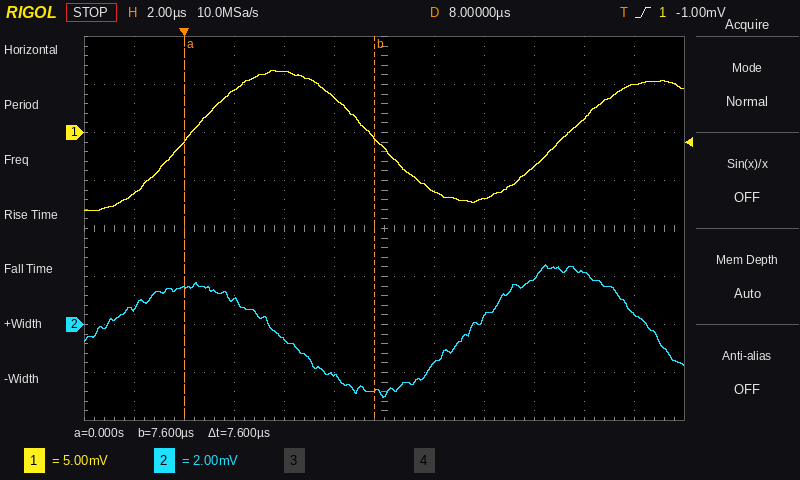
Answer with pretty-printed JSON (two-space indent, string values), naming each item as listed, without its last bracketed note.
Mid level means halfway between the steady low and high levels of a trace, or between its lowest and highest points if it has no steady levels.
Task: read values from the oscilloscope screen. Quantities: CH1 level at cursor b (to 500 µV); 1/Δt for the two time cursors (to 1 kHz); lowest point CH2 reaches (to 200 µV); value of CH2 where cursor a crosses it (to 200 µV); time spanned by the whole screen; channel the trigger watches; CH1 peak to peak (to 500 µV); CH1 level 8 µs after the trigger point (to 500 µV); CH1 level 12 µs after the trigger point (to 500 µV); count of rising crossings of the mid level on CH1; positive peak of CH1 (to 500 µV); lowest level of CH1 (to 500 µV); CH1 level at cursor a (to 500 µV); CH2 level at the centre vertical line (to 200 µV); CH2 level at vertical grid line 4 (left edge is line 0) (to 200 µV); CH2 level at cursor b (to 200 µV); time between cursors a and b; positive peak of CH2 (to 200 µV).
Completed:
{
  "CH1 level at cursor b": "-500 µV",
  "1/Δt for the two time cursors": "132 kHz",
  "lowest point CH2 reaches": "-3.0 mV",
  "value of CH2 where cursor a crosses it": "1.6 mV",
  "time spanned by the whole screen": "24 µs",
  "channel the trigger watches": "CH1",
  "CH1 peak to peak": "14.5 mV",
  "CH1 level 8 µs after the trigger point": "-1.5 mV",
  "CH1 level 12 µs after the trigger point": "-7.0 mV",
  "count of rising crossings of the mid level on CH1": "2",
  "positive peak of CH1": "6.5 mV",
  "lowest level of CH1": "-8.0 mV",
  "CH1 level at cursor a": "-1.0 mV",
  "CH2 level at the centre vertical line": "-3.0 mV",
  "CH2 level at vertical grid line 4 (left edge is line 0)": "-600 µV",
  "CH2 level at cursor b": "-2.8 mV",
  "time between cursors a and b": "7.6 µs",
  "positive peak of CH2": "2.4 mV"
}
